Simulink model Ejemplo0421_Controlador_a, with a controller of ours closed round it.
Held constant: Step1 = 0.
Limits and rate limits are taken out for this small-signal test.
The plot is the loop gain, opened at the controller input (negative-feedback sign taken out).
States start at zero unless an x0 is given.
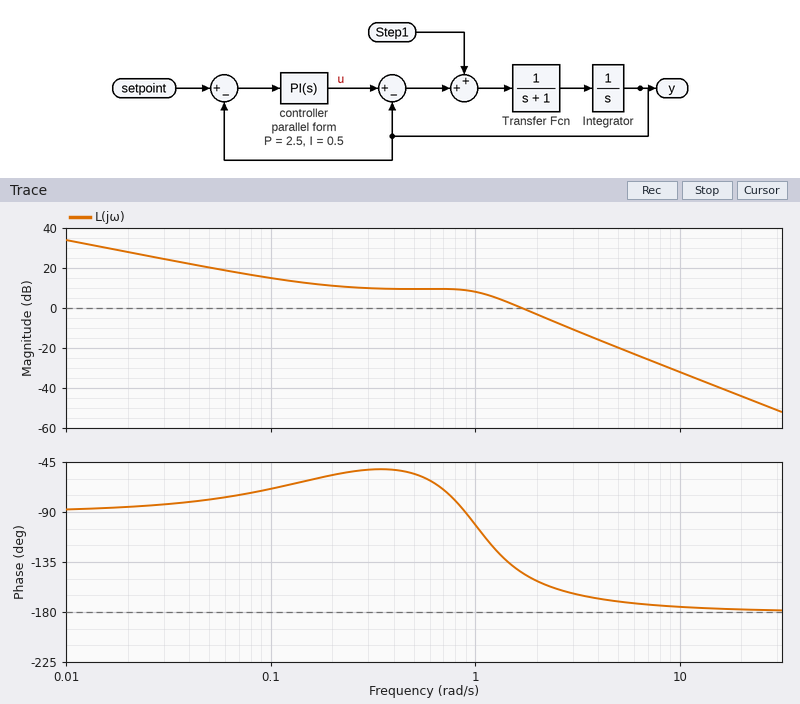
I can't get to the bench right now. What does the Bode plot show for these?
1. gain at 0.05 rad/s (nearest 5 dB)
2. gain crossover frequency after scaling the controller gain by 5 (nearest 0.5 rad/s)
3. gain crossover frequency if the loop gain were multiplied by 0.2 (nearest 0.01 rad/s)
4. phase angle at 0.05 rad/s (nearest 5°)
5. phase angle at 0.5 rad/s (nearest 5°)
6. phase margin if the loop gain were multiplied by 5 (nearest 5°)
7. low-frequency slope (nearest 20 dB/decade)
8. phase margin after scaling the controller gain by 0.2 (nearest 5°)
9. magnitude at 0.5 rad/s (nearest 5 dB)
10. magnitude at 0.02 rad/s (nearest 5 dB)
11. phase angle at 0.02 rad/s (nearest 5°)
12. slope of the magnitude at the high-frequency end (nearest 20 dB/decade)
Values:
20 dB
3.5 rad/s
0.12 rad/s
-80°
-55°
15°
-20 dB/decade
115°
10 dB
30 dB
-85°
-40 dB/decade
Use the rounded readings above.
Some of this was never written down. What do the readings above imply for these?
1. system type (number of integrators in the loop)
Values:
1
